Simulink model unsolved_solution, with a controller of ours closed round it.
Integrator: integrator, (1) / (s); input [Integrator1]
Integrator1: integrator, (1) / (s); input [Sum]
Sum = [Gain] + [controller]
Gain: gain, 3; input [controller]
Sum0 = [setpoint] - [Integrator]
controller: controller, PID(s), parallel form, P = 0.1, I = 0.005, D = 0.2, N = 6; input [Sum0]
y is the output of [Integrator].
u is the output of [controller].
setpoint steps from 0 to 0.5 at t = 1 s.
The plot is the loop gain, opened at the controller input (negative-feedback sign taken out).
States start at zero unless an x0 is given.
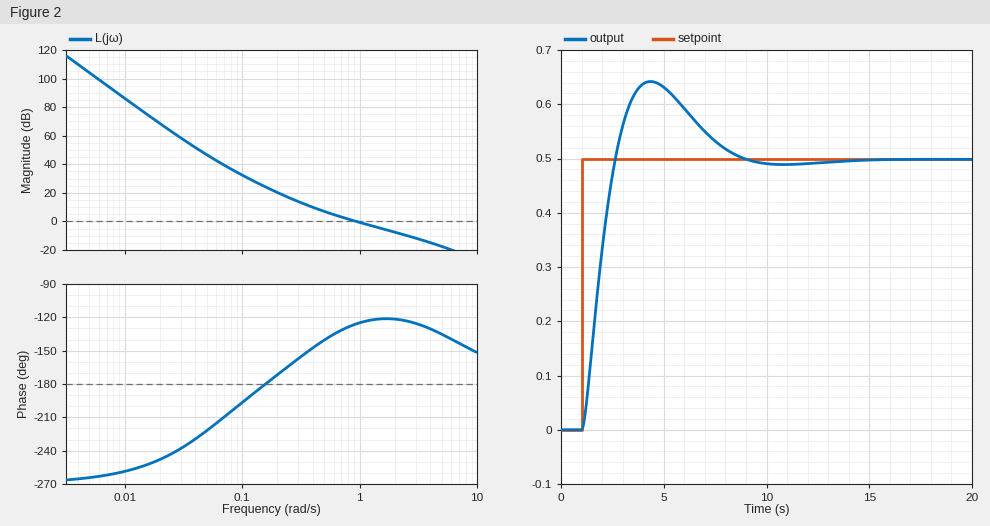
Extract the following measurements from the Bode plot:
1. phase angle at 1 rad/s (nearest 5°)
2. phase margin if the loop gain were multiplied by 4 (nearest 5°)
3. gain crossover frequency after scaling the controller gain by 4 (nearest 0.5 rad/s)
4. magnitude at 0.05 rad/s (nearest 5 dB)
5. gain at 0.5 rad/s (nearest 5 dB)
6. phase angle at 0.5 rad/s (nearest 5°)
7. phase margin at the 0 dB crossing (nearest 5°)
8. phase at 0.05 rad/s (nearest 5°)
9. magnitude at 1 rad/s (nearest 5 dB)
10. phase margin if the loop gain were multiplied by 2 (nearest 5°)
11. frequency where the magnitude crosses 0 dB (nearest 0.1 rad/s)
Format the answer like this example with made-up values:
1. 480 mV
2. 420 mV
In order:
1. -125°
2. 55°
3. 3.0 rad/s
4. 45 dB
5. 5 dB
6. -140°
7. 55°
8. -220°
9. 0 dB
10. 60°
11. 0.9 rad/s
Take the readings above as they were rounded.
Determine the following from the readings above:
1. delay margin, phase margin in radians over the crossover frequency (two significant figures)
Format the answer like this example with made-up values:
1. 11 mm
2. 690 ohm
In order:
1. 1.1 s
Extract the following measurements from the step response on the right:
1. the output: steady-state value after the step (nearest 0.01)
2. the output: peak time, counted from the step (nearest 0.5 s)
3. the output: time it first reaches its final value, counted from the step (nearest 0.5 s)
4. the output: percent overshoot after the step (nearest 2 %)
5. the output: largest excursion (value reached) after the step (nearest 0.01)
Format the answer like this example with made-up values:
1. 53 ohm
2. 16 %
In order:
1. 0.50
2. 3.5 s
3. 1.5 s
4. 28 %
5. 0.64
